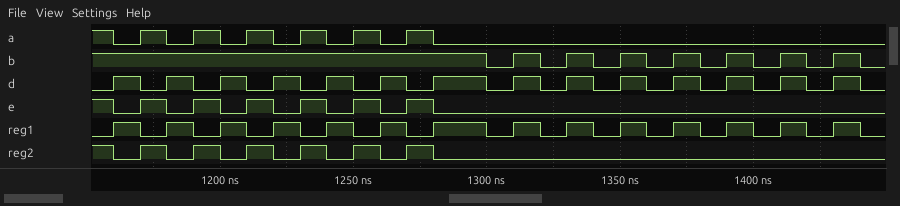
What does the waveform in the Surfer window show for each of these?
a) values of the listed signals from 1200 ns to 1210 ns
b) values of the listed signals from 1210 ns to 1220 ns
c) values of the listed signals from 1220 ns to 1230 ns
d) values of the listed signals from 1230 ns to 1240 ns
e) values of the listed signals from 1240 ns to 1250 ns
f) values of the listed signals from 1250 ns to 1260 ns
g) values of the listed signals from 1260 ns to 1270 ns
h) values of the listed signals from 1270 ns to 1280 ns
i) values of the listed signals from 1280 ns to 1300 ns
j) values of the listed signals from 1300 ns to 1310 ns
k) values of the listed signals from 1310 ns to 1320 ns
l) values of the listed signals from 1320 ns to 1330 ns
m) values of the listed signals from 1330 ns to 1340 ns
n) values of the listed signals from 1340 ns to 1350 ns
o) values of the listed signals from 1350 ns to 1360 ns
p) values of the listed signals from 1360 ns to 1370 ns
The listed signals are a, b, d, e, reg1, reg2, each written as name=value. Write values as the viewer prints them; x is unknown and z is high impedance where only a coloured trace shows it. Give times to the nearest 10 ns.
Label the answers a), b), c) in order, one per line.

a) a=0, b=1, d=1, e=0, reg1=1, reg2=0
b) a=1, b=1, d=0, e=1, reg1=0, reg2=1
c) a=0, b=1, d=1, e=0, reg1=1, reg2=0
d) a=1, b=1, d=0, e=1, reg1=0, reg2=1
e) a=0, b=1, d=1, e=0, reg1=1, reg2=0
f) a=1, b=1, d=0, e=1, reg1=0, reg2=1
g) a=0, b=1, d=1, e=0, reg1=1, reg2=0
h) a=1, b=1, d=0, e=1, reg1=0, reg2=1
i) a=0, b=1, d=1, e=0, reg1=1, reg2=0
j) a=0, b=0, d=0, e=0, reg1=0, reg2=0
k) a=0, b=1, d=1, e=0, reg1=1, reg2=0
l) a=0, b=0, d=0, e=0, reg1=0, reg2=0
m) a=0, b=1, d=1, e=0, reg1=1, reg2=0
n) a=0, b=0, d=0, e=0, reg1=0, reg2=0
o) a=0, b=1, d=1, e=0, reg1=1, reg2=0
p) a=0, b=0, d=0, e=0, reg1=0, reg2=0
